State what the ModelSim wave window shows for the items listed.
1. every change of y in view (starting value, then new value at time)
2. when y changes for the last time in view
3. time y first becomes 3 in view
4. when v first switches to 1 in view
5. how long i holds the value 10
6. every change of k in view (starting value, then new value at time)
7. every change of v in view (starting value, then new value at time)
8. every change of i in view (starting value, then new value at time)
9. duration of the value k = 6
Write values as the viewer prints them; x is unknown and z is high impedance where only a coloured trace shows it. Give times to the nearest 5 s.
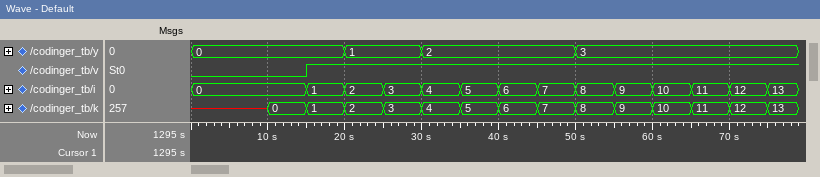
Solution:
0, 1 at 20 s, 2 at 30 s, 3 at 50 s
50 s
50 s
15 s
5 s
x, 0 at 10 s, 1 at 15 s, 2 at 20 s, 3 at 25 s, 4 at 30 s, 5 at 35 s, 6 at 40 s, 7 at 45 s, 8 at 50 s, 9 at 55 s, 10 at 60 s, 11 at 65 s, 12 at 70 s, 13 at 75 s
0, 1 at 15 s
0, 1 at 15 s, 2 at 20 s, 3 at 25 s, 4 at 30 s, 5 at 35 s, 6 at 40 s, 7 at 45 s, 8 at 50 s, 9 at 55 s, 10 at 60 s, 11 at 65 s, 12 at 70 s, 13 at 75 s
5 s
